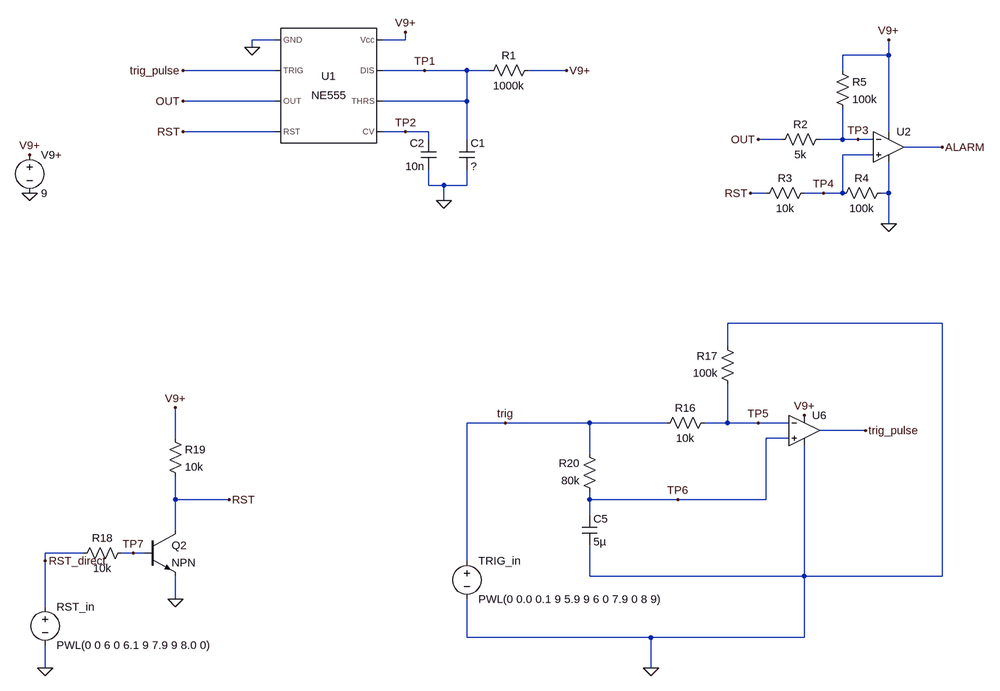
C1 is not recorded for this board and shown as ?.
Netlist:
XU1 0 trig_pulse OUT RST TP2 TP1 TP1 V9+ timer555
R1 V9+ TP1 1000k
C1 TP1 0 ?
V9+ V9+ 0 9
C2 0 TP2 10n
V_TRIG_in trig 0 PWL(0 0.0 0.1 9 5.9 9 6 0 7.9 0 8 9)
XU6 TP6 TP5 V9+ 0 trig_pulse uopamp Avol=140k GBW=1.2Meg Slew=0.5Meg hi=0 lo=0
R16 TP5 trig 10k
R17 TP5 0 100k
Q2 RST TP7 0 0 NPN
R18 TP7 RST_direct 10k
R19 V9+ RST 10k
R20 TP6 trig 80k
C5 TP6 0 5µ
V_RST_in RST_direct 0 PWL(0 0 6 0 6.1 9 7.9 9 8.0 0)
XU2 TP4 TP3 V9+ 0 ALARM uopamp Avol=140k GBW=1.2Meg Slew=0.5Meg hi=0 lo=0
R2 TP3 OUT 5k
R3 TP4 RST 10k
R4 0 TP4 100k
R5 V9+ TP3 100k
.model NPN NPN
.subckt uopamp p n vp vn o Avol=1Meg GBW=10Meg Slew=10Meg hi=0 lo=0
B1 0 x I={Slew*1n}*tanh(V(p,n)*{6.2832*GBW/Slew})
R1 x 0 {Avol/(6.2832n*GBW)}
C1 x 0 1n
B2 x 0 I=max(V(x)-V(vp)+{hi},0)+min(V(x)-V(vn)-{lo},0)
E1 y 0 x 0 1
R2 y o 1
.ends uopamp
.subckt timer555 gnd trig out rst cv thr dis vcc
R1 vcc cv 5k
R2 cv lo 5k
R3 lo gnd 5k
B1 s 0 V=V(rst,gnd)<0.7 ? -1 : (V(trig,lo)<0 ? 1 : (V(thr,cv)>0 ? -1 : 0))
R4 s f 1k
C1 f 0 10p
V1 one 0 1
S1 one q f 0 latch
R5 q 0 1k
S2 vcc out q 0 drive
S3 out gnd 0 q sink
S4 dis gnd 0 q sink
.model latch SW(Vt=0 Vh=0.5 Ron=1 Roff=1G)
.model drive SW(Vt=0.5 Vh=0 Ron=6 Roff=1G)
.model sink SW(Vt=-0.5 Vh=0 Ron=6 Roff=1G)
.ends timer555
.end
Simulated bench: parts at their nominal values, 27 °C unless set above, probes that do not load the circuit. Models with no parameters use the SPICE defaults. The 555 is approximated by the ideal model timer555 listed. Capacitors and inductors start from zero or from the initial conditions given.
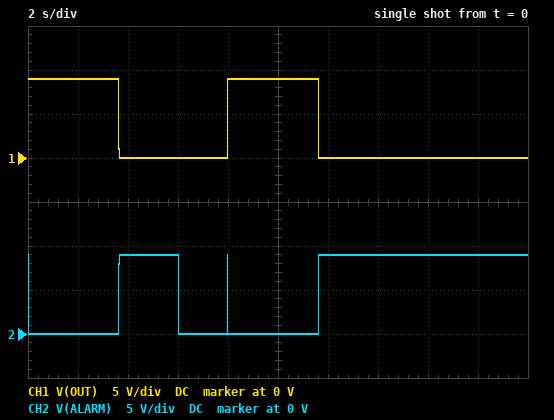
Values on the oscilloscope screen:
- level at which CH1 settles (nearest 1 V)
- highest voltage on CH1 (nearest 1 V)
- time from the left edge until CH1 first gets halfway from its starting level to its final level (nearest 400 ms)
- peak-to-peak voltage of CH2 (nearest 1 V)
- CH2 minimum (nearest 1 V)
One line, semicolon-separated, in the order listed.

0 V; 9 V; 3.6 s; 9 V; 0 V
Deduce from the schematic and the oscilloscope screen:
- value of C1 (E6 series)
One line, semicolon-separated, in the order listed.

3.3 µF
